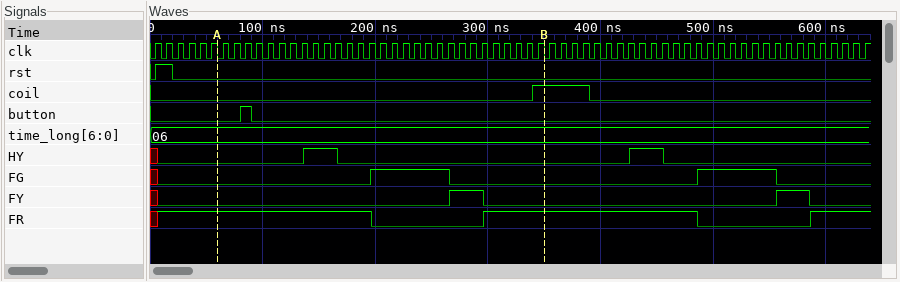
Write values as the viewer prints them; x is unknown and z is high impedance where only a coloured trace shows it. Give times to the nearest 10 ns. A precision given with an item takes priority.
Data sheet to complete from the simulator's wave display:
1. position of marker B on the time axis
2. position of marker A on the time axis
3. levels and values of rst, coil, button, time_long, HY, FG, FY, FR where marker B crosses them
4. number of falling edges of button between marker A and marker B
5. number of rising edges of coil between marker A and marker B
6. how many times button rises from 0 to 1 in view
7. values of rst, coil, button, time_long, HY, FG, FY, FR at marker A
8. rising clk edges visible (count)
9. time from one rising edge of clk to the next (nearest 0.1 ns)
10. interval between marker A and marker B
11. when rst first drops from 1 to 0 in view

350 ns
60 ns
rst=0, coil=1, button=0, time_long=06, HY=0, FG=0, FY=0, FR=1
1
1
1
rst=0, coil=0, button=0, time_long=06, HY=0, FG=0, FY=0, FR=1
64
10 ns
290 ns
20 ns
